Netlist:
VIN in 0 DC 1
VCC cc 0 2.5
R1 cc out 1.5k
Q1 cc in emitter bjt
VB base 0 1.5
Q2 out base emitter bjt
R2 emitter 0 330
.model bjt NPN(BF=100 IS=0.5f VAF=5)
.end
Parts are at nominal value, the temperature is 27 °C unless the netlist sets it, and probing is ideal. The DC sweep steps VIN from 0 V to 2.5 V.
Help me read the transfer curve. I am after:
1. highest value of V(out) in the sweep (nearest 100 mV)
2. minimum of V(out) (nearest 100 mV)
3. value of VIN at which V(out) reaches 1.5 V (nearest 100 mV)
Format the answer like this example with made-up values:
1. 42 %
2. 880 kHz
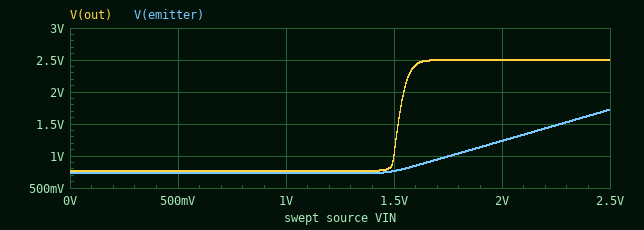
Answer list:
1. 2.5 V
2. 800 mV
3. 1.5 V
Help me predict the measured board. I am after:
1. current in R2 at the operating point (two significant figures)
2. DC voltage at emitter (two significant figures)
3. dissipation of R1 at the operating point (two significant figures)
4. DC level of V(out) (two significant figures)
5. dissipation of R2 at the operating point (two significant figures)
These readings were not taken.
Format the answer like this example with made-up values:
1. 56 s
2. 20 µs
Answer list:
1. 2.2 mA
2. 730 mV
3. 2.0 mW
4. 770 mV
5. 1.6 mW
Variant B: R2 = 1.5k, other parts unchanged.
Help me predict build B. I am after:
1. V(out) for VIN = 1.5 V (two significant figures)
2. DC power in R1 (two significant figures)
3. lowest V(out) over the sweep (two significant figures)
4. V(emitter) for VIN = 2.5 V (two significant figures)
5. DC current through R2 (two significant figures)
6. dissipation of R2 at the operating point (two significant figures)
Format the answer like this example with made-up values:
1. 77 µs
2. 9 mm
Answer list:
1. 2.1 V
2. 400 µW
3. 1.7 V
4. 1.8 V
5. 520 µA
6. 410 µW
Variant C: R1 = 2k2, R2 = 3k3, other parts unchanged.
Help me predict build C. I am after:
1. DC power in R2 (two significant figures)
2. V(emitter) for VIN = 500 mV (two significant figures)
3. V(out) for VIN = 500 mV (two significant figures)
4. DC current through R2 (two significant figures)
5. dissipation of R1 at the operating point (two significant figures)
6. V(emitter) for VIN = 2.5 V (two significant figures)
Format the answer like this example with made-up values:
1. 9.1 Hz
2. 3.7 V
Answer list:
1. 200 µW
2. 810 mV
3. 2.0 V
4. 240 µA
5. 130 µW
6. 1.8 V
